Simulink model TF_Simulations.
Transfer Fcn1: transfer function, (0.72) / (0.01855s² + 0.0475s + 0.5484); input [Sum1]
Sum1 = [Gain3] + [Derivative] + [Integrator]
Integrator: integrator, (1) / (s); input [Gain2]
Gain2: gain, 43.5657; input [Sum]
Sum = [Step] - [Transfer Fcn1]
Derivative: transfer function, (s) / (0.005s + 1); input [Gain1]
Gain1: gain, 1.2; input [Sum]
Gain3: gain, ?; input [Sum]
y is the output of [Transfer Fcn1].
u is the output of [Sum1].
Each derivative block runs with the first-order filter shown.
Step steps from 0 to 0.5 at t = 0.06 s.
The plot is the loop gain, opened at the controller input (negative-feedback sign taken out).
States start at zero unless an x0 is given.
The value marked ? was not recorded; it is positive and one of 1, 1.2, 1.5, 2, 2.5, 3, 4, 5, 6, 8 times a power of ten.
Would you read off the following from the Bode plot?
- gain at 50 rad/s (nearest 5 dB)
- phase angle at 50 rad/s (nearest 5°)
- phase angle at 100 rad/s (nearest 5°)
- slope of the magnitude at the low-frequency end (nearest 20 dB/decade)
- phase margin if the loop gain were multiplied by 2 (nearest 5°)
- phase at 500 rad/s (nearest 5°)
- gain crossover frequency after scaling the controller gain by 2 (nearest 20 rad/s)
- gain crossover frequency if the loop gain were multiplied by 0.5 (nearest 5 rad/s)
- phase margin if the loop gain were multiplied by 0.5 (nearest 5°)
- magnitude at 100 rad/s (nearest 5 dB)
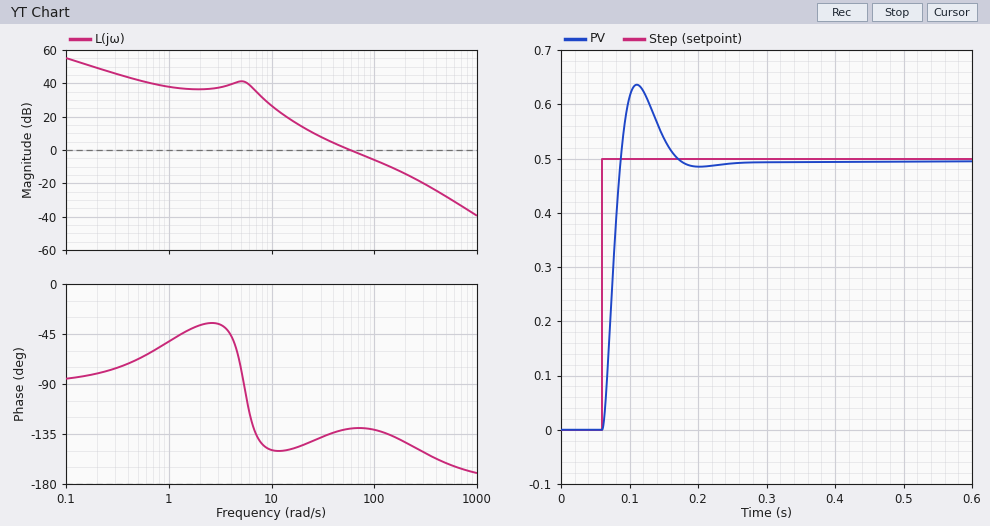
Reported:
0 dB
-130°
-130°
-20 dB/decade
50°
-160°
100 rad/s
35 rad/s
45°
-5 dB
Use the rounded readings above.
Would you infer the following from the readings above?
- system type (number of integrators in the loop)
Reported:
1
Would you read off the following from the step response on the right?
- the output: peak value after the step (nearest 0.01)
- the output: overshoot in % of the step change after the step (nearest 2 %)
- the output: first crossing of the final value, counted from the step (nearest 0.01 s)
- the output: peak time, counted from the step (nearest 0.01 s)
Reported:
0.64
28 %
0.03 s
0.05 s
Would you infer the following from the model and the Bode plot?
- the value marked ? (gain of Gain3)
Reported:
40
